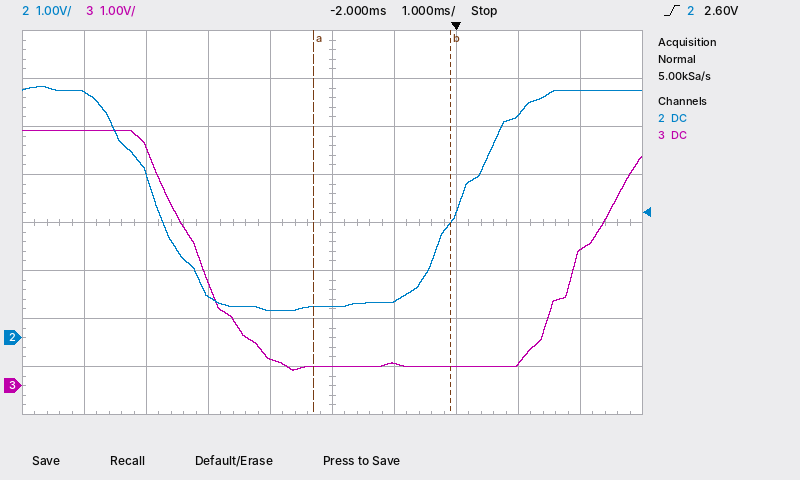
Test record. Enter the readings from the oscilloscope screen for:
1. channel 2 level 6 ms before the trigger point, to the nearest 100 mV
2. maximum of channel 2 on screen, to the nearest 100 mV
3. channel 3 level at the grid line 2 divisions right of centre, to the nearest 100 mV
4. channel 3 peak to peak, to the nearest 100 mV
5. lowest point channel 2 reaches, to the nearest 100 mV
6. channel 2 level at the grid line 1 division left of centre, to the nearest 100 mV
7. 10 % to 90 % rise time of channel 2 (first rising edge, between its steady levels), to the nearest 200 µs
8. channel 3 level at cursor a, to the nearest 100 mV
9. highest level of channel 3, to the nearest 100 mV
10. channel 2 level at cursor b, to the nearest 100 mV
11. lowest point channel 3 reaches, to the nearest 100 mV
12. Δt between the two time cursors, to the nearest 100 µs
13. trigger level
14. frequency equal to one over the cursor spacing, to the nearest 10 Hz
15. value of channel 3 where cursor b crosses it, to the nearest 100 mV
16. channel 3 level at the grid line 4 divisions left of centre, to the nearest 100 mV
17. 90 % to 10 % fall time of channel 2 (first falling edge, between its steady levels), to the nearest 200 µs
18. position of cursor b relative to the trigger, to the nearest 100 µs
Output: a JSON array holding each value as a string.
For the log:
["5.1 V", "5.2 V", "400 mV", "5.0 V", "600 mV", "600 mV", "1.6 ms", "400 mV", "5.3 V", "2.4 V", "300 mV", "2.2 ms", "2.60 V", "450 Hz", "400 mV", "5.3 V", "1.6 ms", "-100 µs"]
